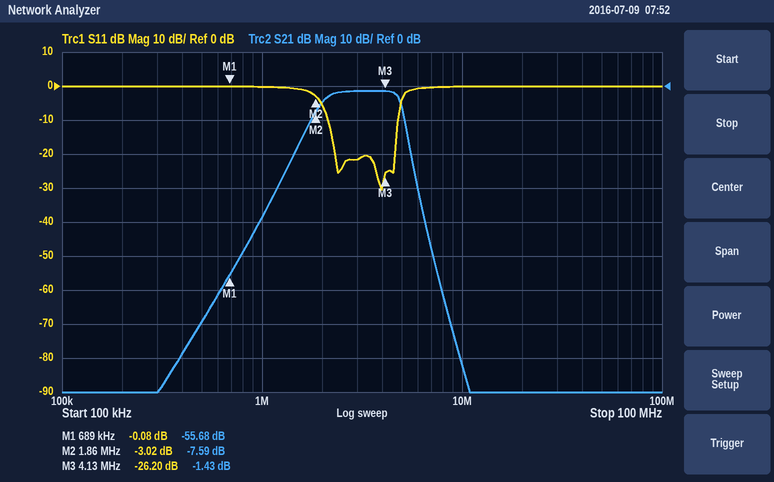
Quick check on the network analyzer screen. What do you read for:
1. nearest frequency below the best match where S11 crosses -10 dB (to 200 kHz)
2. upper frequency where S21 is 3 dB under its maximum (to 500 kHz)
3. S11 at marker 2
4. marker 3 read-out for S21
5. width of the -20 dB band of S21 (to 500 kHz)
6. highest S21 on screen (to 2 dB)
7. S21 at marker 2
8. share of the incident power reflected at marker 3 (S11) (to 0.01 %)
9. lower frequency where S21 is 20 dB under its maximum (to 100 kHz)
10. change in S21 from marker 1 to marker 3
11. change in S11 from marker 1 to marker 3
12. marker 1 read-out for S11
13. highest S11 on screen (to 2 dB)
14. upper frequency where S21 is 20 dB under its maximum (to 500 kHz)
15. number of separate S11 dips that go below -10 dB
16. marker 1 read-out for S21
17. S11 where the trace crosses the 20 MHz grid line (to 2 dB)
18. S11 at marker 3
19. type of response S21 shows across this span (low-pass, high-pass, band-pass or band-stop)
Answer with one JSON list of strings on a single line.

["2.2 MHz", "5.0 MHz", "-3.02 dB", "-1.43 dB", "4.0 MHz", "-2 dB", "-7.59 dB", "0.24 %", "1.4 MHz", "54.25 dB", "-26.12 dB", "-0.08 dB", "0 dB", "5.5 MHz", "2", "-55.68 dB", "0 dB", "-26.20 dB", "band-pass"]
